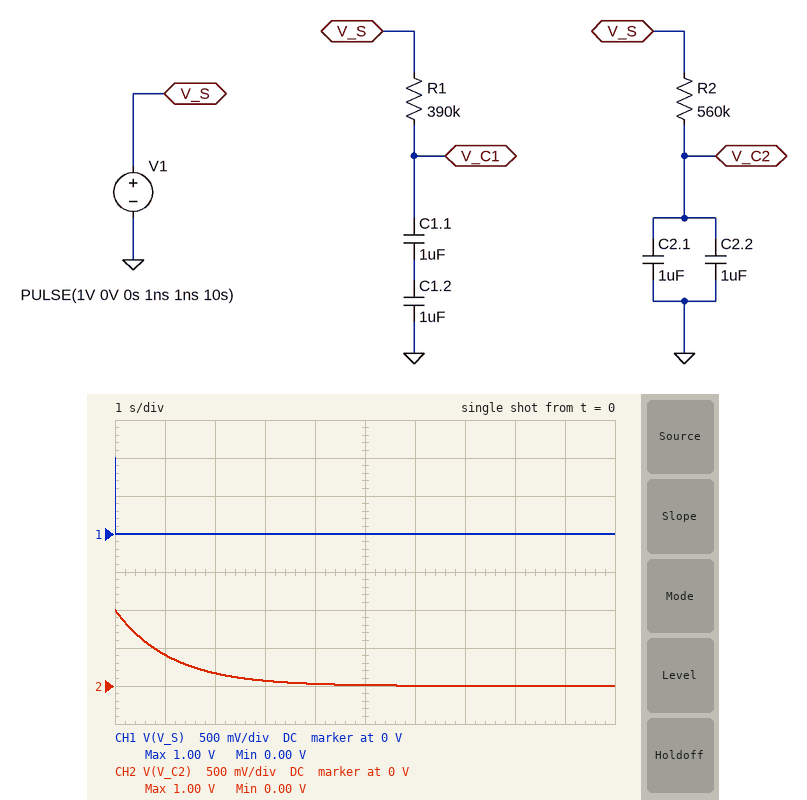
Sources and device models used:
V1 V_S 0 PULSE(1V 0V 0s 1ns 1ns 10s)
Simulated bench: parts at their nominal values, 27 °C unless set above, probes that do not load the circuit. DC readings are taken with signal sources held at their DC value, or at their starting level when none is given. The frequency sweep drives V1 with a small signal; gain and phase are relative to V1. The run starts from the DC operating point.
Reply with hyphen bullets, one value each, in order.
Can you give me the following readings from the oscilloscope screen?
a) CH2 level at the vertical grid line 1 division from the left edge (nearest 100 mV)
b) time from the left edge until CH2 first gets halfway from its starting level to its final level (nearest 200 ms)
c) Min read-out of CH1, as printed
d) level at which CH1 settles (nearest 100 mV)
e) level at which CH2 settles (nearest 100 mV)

- 400 mV
- 800 ms
- 0.00 V
- 0 V
- 0 V
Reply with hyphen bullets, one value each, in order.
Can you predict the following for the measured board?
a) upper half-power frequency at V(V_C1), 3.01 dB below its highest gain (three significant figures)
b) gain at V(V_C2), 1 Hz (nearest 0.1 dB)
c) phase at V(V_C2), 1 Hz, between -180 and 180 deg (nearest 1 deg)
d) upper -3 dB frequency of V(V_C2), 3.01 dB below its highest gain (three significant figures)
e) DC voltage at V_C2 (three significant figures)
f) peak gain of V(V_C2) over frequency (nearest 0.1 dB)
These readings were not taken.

- 816 mHz
- -17.0 dB
- -82 deg
- 142 mHz
- 1.00 V
- 0 dB
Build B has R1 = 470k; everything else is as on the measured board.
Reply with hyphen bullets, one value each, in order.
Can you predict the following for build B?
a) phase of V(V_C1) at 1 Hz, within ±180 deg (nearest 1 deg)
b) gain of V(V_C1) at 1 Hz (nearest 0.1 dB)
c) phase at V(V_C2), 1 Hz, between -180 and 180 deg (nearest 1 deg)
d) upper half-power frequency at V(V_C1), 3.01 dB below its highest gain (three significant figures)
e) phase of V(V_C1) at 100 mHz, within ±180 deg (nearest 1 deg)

- -56 deg
- -5.0 dB
- -82 deg
- 677 mHz
- -8 deg
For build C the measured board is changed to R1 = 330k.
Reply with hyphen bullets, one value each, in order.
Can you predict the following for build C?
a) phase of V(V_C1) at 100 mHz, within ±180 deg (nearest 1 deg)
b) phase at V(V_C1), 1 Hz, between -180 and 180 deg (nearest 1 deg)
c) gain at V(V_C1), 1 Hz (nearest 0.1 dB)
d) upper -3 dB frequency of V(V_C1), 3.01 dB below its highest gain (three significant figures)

- -6 deg
- -46 deg
- -3.2 dB
- 965 mHz
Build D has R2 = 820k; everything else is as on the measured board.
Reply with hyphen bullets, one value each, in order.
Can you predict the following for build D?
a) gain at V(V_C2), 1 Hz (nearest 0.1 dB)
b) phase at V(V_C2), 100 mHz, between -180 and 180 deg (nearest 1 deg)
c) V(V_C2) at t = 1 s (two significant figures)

- -20.3 dB
- -46 deg
- 540 mV
